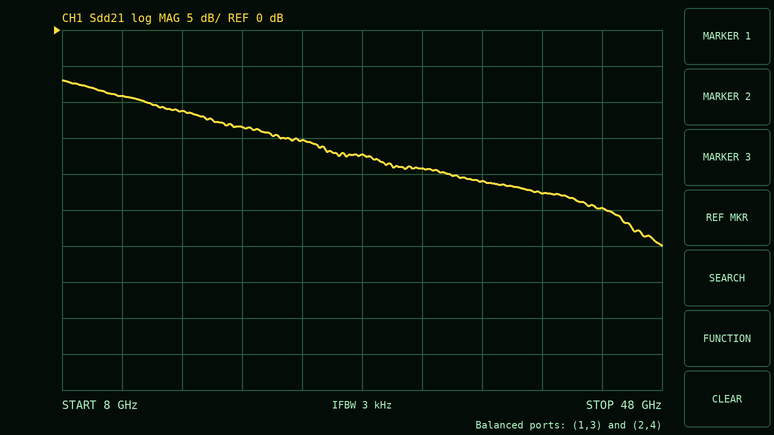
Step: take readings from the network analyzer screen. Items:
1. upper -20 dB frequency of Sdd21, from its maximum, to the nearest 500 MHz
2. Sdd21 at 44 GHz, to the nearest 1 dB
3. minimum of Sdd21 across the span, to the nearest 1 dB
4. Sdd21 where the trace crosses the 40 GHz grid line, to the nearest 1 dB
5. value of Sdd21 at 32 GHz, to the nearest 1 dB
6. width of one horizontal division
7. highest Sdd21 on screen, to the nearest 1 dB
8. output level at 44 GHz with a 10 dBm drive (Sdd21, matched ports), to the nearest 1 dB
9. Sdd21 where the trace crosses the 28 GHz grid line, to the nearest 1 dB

46.0 GHz
-25 dB
-30 dB
-23 dB
-19 dB
4 GHz
-7 dB
-15 dBm
-17 dB
